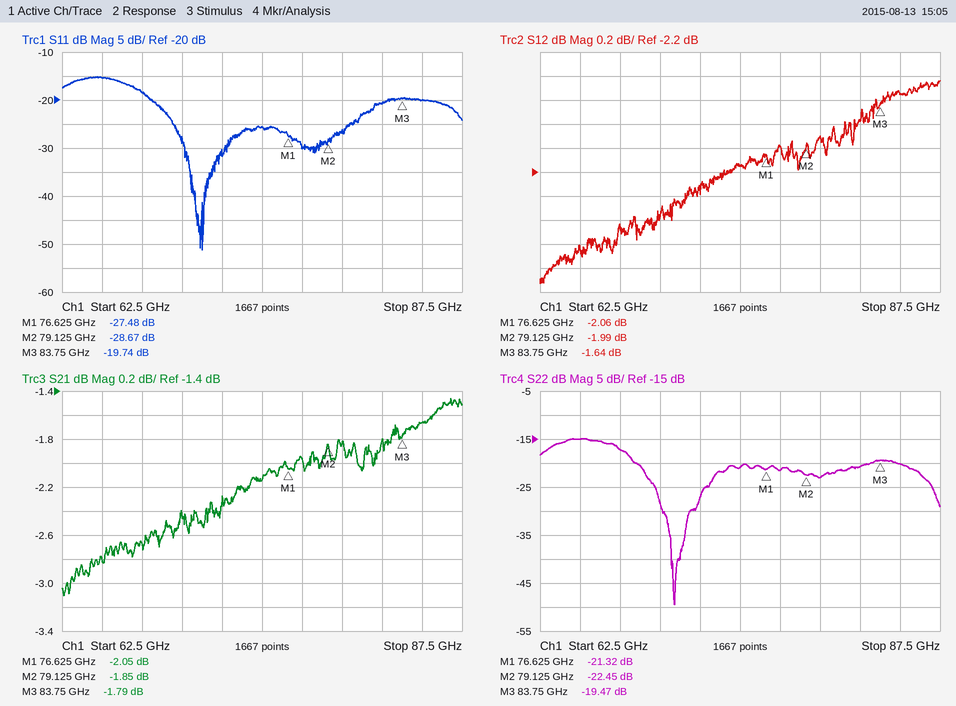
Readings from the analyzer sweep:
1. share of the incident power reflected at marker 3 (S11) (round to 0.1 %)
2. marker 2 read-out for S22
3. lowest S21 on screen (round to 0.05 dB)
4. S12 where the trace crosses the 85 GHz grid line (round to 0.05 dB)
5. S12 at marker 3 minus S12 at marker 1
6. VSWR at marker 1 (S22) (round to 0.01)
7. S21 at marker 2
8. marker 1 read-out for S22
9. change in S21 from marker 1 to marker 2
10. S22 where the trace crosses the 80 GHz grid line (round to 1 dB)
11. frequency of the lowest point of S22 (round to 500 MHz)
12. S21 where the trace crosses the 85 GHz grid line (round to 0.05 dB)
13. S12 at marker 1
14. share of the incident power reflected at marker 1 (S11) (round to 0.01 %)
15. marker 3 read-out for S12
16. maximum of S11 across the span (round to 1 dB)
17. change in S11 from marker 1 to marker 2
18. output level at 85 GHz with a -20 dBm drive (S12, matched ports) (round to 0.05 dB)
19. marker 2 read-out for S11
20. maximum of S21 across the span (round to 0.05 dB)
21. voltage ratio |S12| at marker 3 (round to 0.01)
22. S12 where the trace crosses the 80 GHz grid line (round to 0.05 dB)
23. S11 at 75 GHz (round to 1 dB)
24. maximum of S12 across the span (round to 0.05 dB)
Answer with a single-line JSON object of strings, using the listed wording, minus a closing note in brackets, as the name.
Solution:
{"share of the incident power reflected at marker 3 (S11)": "1.1 %", "marker 2 read-out for S22": "-22.45 dB", "lowest S21 on screen": "-3.10 dB", "S12 where the trace crosses the 85 GHz grid line": "-1.55 dB", "S12 at marker 3 minus S12 at marker 1": "0.42 dB", "VSWR at marker 1 (S22)": "1.19", "S21 at marker 2": "-1.85 dB", "marker 1 read-out for S22": "-21.32 dB", "change in S21 from marker 1 to marker 2": "0.20 dB", "S22 where the trace crosses the 80 GHz grid line": "-23 dB", "frequency of the lowest point of S22": "71.0 GHz", "S21 where the trace crosses the 85 GHz grid line": "-1.65 dB", "S12 at marker 1": "-2.06 dB", "share of the incident power reflected at marker 1 (S11)": "0.18 %", "marker 3 read-out for S12": "-1.64 dB", "maximum of S11 across the span": "-15 dB", "change in S11 from marker 1 to marker 2": "-1.19 dB", "output level at 85 GHz with a -20 dBm drive (S12, matched ports)": "-21.55 dBm", "marker 2 read-out for S11": "-28.67 dB", "maximum of S21 across the span": "-1.45 dB", "voltage ratio |S12| at marker 3": "0.83", "S12 where the trace crosses the 80 GHz grid line": "-1.90 dB", "S11 at 75 GHz": "-26 dB", "maximum of S12 across the span": "-1.45 dB"}
